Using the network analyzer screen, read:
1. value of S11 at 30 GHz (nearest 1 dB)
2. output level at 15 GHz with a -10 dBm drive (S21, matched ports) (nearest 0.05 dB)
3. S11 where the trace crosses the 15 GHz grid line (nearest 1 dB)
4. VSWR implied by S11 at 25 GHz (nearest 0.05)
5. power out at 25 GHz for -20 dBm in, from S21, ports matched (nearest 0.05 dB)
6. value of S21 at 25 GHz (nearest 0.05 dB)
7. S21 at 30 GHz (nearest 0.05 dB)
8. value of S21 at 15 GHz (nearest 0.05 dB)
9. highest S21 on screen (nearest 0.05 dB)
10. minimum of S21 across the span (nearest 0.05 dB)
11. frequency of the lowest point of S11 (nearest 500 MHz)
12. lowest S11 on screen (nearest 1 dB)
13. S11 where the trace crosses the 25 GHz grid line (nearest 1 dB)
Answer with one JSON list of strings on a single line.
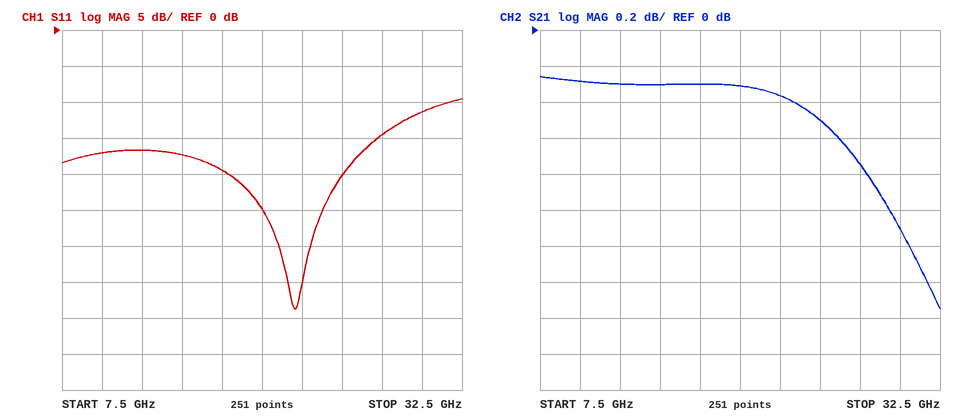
["-11 dB", "-10.30 dBm", "-17 dB", "1.20", "-20.50 dBm", "-0.50 dB", "-1.10 dB", "-0.30 dB", "-0.25 dB", "-1.55 dB", "22.0 GHz", "-39 dB", "-20 dB"]
